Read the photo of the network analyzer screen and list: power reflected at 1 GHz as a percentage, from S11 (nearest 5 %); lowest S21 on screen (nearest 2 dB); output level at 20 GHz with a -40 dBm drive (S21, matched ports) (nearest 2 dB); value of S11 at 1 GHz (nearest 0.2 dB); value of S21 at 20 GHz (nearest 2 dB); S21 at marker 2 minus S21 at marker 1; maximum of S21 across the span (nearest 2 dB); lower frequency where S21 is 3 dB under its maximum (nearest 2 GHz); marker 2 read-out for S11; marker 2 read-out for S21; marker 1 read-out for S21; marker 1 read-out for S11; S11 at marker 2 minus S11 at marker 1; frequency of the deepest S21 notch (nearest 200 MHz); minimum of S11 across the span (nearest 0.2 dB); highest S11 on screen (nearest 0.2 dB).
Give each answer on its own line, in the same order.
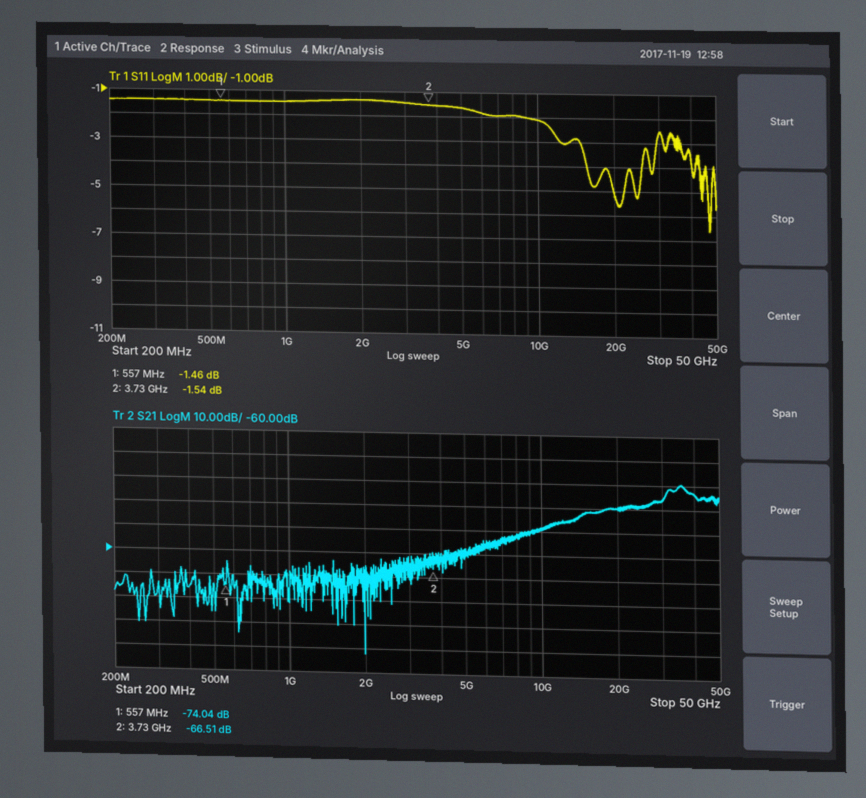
70 %
-102 dB
-80 dBm
-1.4 dB
-40 dB
7.53 dB
-30 dB
32 GHz
-1.54 dB
-66.51 dB
-74.04 dB
-1.46 dB
-0.08 dB
2.0 GHz
-6.6 dB
-1.4 dB
